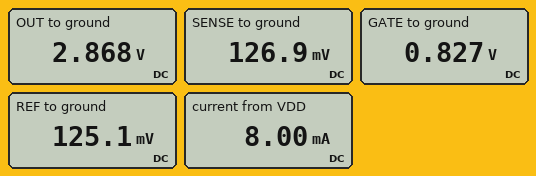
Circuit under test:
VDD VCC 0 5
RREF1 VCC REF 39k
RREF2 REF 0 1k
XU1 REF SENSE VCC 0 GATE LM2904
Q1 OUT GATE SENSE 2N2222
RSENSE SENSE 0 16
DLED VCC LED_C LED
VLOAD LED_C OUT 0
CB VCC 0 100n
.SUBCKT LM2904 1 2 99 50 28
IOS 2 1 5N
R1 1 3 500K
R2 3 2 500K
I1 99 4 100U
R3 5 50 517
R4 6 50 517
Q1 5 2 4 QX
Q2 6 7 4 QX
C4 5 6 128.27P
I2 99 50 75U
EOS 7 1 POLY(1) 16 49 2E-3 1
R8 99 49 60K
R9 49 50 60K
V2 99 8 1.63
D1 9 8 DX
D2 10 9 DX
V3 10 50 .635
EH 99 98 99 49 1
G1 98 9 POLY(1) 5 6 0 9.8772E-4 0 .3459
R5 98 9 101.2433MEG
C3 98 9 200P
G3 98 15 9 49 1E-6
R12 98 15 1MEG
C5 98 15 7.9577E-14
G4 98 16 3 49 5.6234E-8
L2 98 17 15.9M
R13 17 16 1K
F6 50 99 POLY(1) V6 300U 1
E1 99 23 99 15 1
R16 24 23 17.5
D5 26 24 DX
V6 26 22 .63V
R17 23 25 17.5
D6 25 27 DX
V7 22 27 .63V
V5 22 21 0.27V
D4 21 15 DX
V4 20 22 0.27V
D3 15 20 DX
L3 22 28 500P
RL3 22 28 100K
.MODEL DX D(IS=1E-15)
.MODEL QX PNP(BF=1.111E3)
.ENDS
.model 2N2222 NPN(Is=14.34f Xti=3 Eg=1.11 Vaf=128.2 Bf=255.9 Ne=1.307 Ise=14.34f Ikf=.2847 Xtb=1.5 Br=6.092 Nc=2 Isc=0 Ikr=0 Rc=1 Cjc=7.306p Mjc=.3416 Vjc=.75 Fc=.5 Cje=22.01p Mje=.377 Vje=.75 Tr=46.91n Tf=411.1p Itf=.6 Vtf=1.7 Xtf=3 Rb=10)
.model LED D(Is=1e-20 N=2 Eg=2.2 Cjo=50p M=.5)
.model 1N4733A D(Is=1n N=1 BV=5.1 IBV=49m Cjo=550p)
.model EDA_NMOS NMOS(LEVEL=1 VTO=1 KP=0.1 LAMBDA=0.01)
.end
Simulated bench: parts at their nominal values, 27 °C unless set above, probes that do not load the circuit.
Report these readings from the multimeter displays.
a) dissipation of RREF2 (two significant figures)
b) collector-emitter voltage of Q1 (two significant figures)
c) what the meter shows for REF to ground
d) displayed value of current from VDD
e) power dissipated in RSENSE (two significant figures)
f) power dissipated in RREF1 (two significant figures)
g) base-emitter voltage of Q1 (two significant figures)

16 µW
2.7 V
125.1 mV
8.00 mA
1.0 mW
610 µW
700 mV
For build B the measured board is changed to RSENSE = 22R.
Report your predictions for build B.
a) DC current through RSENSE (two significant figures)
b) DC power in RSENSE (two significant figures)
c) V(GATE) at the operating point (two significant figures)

5.8 mA
730 µW
820 mV
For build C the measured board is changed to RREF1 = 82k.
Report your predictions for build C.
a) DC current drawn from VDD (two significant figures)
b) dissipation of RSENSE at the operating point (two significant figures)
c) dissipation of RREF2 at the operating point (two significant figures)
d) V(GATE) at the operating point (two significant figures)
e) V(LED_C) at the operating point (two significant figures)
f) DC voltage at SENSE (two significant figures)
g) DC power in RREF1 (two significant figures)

3.9 mA
240 µW
3.6 µW
740 mV
2.9 V
62 mV
300 µW
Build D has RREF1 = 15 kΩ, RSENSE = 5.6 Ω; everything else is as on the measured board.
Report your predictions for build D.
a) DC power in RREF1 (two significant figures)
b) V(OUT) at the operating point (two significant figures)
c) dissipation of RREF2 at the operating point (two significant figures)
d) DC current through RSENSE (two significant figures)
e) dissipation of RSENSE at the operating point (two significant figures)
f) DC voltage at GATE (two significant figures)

1.5 mW
2.8 V
98 µW
56 mA
18 mW
1.1 V
